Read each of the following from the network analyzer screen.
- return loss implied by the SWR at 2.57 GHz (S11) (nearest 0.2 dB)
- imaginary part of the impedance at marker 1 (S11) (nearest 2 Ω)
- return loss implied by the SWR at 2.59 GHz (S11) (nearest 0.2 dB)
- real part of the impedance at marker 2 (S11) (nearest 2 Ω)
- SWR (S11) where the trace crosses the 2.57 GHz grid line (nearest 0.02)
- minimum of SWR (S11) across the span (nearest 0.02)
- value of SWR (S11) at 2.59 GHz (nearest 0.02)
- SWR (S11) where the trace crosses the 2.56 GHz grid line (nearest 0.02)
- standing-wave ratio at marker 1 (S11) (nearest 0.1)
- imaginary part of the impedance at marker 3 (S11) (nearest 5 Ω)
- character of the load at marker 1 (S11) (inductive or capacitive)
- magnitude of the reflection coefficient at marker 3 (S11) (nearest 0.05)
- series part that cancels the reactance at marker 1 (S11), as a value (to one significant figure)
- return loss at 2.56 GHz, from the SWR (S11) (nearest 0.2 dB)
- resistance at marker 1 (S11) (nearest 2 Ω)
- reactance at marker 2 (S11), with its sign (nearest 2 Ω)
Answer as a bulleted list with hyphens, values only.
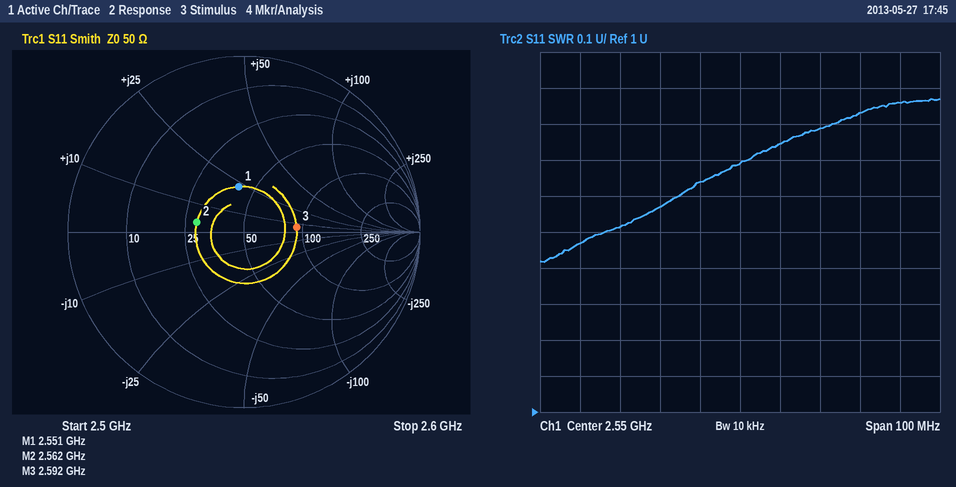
- 11.0 dB
- +22 Ω
- 10.4 dB
- 28 Ω
- 1.78
- 1.42
- 1.86
- 1.74
- 1.7
- +5 Ω
- inductive
- 0.30
- 3 pF
- 11.4 dB
- 42 Ω
- +4 Ω
